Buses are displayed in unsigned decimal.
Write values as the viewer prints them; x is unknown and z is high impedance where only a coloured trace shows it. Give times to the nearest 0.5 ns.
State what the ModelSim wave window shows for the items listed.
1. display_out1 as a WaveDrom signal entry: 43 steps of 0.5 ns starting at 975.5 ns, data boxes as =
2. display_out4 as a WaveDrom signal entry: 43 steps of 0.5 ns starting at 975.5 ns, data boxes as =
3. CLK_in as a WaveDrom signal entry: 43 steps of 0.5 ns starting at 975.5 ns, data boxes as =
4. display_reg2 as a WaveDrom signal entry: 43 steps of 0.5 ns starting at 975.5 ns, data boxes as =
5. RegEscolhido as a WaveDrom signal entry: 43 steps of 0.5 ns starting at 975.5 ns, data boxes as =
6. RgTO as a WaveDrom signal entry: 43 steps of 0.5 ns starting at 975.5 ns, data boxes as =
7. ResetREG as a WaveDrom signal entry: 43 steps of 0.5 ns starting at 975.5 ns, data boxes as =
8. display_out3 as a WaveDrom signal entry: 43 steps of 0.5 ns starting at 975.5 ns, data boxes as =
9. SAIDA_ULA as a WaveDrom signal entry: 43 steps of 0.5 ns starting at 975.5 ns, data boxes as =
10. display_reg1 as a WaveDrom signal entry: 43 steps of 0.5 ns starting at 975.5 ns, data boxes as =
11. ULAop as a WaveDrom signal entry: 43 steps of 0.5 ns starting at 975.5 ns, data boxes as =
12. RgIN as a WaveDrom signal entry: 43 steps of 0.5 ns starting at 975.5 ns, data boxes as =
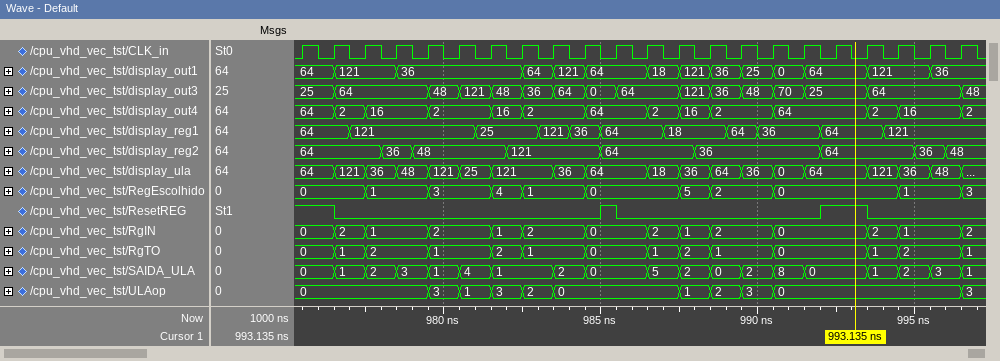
{name: 'display_out1', wave: '=.=...=.......=.=.=...=.=.=.=.=.=...=...=..', data: '64 121 36 64 121 64 18 121 36 25 0 64 121 36'}
{name: 'display_out4', wave: '=.=.=...=...=.=...=...=.=.=...=.....=.=...=', data: '64 2 16 2 16 2 64 2 16 2 64 2 16 2'}
{name: 'CLK_in', wave: '1010101010101010101010101010101010101010101'}
{name: 'display_reg2', wave: '=....=.=.....=.....=.....=.......=.....=.=.', data: '64 36 48 121 64 36 64 36 48'}
{name: 'RegEscolhido', wave: '=...=...=...=.=...=.....=.=...=.......=...=', data: '0 1 3 4 1 0 5 2 0 1 3'}
{name: 'RgTO', wave: '=.=.=...=...=.=...=...=.=.=...=.....=.=...=', data: '0 1 2 1 2 1 0 1 2 1 0 1 2 1'}
{name: 'ResetREG', wave: '1.0................10............1..0......'}
{name: 'display_out3', wave: '=.=.....=.=.=.=.=.=.=...=.=.=.=.=...=.....=', data: '25 64 48 121 48 36 64 0 64 121 36 48 70 25 64 48'}
{name: 'SAIDA_ULA', wave: '=.=.=.=.=.=.=...=.=...=.=.=.=.=.=...=.=.=.=', data: '0 1 2 3 1 4 1 2 0 5 2 0 2 8 0 1 2 3 1'}
{name: 'display_reg1', wave: '=..=.......=...=.=.=...=...=.=...=...=.....', data: '64 121 25 121 36 64 18 64 36 64 121'}
{name: 'ULAop', wave: '=.......=.=.=.=.=.......=.=.=.=...........=', data: '0 3 1 3 2 0 1 2 3 0 3'}
{name: 'RgIN', wave: '=.=.=...=...=.=...=...=.=.=...=.....=.=...=', data: '0 2 1 2 1 2 0 2 1 2 0 2 1 2'}
